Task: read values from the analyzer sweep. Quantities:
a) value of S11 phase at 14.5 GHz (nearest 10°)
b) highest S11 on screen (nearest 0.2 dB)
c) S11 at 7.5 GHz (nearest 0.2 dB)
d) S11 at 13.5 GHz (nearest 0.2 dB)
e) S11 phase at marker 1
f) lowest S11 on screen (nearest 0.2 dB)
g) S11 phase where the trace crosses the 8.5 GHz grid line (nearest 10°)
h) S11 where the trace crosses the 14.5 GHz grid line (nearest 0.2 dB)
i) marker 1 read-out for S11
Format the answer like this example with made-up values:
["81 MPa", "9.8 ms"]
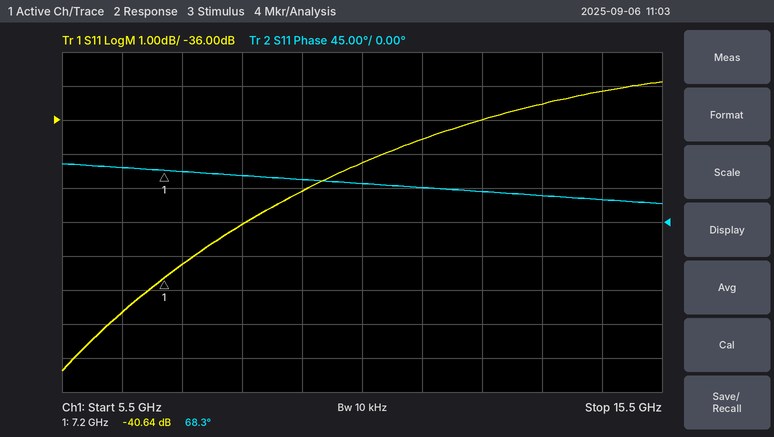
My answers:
["30°", "-34.8 dB", "-40.2 dB", "-35.6 dB", "68.3°", "-43.4 dB", "60°", "-35.2 dB", "-40.64 dB"]
